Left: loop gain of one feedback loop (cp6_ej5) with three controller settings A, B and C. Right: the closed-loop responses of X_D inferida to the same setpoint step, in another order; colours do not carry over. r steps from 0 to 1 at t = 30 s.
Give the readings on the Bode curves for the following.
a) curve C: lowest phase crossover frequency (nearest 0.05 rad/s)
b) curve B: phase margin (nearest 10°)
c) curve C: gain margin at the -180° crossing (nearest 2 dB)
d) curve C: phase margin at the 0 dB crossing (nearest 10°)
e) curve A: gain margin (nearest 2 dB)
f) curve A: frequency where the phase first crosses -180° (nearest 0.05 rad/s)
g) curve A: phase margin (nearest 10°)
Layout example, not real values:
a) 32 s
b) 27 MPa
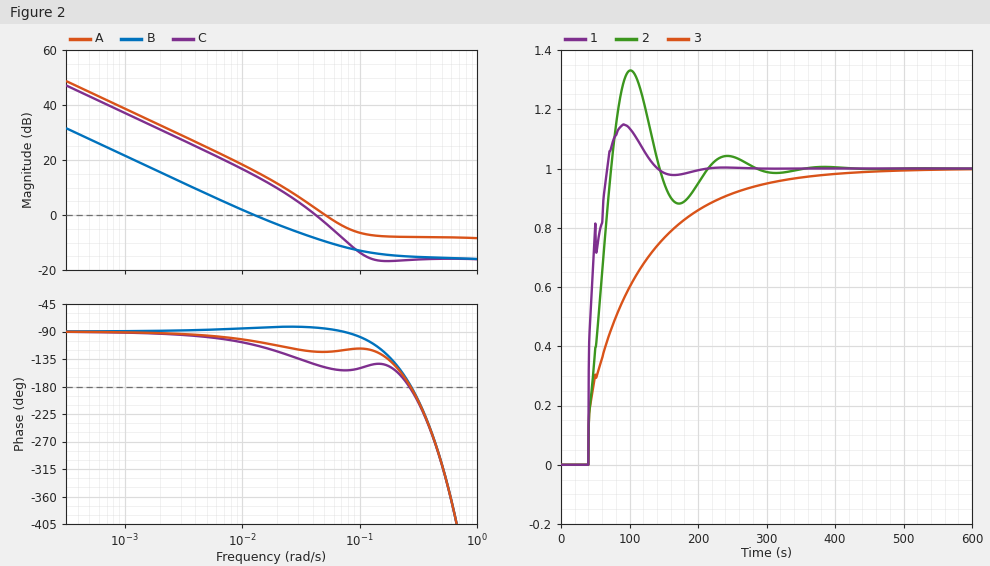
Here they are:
a) 0.25 rad/s
b) 100°
c) 16 dB
d) 40°
e) 8 dB
f) 0.25 rad/s
g) 60°
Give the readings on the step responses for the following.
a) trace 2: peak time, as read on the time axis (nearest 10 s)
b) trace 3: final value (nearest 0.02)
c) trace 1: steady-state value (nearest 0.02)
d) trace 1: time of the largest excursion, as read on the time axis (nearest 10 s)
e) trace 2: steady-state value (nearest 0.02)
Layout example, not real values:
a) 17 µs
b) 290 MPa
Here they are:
a) 100 s
b) 1.00
c) 1.00
d) 90 s
e) 1.00
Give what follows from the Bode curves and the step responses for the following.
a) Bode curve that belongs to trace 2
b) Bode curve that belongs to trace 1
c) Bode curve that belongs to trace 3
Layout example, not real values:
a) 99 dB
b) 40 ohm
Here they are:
a) C
b) A
c) B
